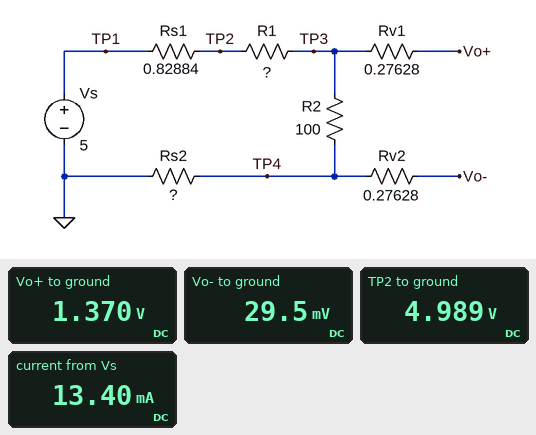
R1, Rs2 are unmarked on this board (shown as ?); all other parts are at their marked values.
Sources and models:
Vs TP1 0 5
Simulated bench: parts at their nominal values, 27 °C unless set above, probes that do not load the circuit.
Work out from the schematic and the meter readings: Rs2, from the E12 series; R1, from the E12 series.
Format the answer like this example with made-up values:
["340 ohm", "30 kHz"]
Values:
["2.2 Ω", "270 Ω"]
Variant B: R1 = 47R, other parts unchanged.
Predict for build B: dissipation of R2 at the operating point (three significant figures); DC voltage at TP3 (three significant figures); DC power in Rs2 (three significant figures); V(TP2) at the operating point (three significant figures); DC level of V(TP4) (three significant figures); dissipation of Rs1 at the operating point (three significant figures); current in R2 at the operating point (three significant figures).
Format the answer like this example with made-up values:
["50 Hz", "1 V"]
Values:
["111 mW", "3.41 V", "2.44 mW", "4.97 V", "73.3 mV", "921 µW", "33.3 mA"]
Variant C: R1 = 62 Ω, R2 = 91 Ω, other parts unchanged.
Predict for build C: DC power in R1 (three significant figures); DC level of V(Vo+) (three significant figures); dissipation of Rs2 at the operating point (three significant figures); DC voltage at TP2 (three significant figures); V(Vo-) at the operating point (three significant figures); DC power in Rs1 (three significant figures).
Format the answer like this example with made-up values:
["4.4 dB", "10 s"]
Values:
["63.7 mW", "2.99 V", "2.26 mW", "4.97 V", "70.5 mV", "851 µW"]
